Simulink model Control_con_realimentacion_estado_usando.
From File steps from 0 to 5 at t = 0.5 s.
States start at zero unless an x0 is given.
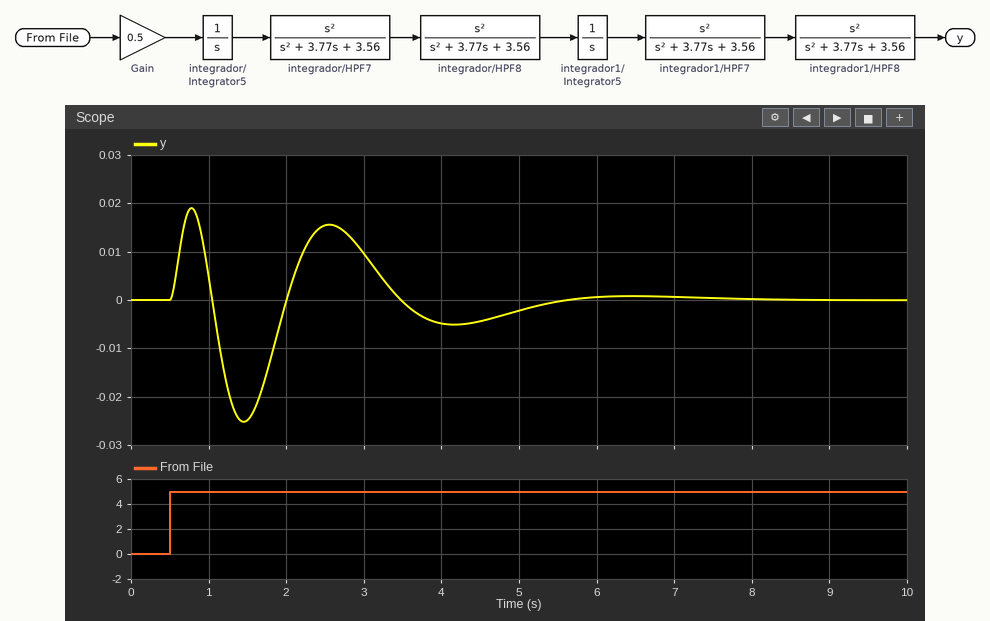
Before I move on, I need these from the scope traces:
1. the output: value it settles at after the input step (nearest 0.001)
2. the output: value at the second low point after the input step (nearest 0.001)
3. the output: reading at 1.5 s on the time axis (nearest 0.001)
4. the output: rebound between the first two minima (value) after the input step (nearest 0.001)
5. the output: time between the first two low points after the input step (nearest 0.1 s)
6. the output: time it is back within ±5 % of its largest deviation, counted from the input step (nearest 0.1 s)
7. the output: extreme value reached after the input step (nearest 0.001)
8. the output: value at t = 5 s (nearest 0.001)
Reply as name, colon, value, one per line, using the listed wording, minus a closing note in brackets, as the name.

the output: value it settles at after the input step: 0.000
the output: value at the second low point after the input step: -0.005
the output: reading at 1.5 s on the time axis: -0.025
the output: rebound between the first two minima (value) after the input step: 0.016
the output: time between the first two low points after the input step: 2.7 s
the output: time it is back within ±5 % of its largest deviation, counted from the input step: 4.7 s
the output: extreme value reached after the input step: -0.025
the output: value at t = 5 s: -0.002
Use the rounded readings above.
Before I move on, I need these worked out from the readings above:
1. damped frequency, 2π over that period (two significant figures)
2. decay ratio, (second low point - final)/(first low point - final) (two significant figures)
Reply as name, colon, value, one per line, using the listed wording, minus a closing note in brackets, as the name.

damped frequency, 2π over that period: 2.3 rad/s
decay ratio, (second low point - final)/(first low point - final): 0.20
